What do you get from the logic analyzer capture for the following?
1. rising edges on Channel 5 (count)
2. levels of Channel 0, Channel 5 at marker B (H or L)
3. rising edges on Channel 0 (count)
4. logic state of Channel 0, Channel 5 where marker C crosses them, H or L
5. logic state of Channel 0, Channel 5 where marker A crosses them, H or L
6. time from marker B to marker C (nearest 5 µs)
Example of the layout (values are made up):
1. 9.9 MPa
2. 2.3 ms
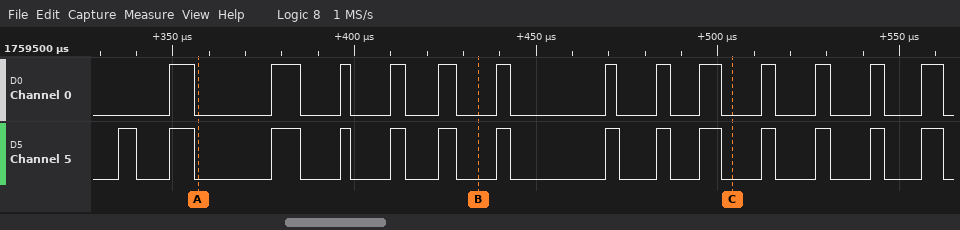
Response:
1. 14
2. Channel 0=L, Channel 5=L
3. 13
4. Channel 0=L, Channel 5=L
5. Channel 0=L, Channel 5=L
6. 70 µs
